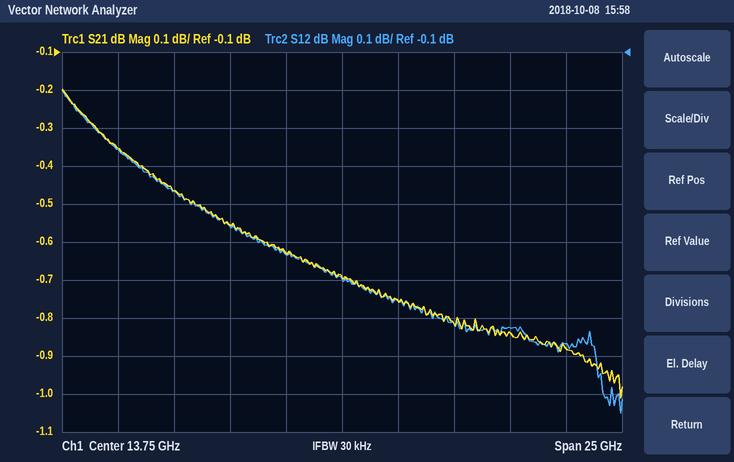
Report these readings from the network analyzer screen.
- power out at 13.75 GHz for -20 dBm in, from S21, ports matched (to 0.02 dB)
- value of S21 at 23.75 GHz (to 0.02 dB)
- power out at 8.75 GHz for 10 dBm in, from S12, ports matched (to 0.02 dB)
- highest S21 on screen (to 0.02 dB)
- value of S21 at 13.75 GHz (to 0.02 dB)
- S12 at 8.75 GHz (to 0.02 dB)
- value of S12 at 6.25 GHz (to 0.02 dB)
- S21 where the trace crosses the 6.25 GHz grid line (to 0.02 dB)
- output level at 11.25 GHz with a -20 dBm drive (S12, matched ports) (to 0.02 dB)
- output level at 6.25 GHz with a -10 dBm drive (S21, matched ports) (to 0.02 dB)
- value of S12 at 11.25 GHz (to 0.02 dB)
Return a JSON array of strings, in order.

["-20.70 dBm", "-0.88 dB", "9.44 dBm", "-0.20 dB", "-0.70 dB", "-0.56 dB", "-0.46 dB", "-0.46 dB", "-20.64 dBm", "-10.46 dBm", "-0.64 dB"]
